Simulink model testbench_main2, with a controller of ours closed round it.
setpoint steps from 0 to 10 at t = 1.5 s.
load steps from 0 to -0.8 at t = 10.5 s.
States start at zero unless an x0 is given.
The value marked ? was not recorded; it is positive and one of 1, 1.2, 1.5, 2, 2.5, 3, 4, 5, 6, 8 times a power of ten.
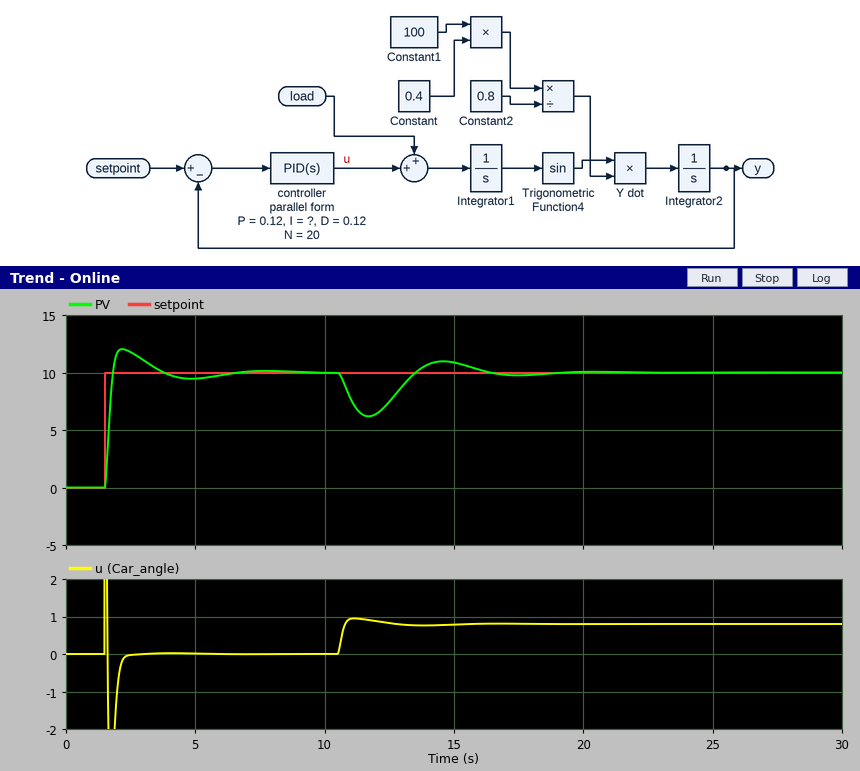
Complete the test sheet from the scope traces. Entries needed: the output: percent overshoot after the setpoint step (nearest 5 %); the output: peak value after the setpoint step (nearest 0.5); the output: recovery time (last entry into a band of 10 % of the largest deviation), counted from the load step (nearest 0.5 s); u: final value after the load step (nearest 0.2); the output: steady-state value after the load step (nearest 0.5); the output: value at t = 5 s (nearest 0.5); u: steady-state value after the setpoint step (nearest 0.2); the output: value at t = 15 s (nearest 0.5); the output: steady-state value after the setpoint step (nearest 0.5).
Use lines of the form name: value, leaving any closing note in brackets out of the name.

the output: percent overshoot after the setpoint step: 20 %
the output: peak value after the setpoint step: 12.0
the output: recovery time (last entry into a band of 10 % of the largest deviation), counted from the load step: 5.5 s
u: final value after the load step: 0.8
the output: steady-state value after the load step: 10.0
the output: value at t = 5 s: 9.5
u: steady-state value after the setpoint step: 0.0
the output: value at t = 15 s: 11.0
the output: steady-state value after the setpoint step: 10.0
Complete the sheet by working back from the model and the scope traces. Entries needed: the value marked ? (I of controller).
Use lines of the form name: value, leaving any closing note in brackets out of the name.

the value marked ?: 0.15
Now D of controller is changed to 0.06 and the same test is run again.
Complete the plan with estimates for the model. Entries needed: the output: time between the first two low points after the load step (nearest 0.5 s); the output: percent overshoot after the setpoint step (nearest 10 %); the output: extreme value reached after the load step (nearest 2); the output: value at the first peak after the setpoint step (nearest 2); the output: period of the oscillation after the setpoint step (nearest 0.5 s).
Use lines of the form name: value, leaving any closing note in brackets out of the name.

the output: time between the first two low points after the load step: 3.5 s
the output: percent overshoot after the setpoint step: 50 %
the output: extreme value reached after the load step: 4
the output: value at the first peak after the setpoint step: 14
the output: period of the oscillation after the setpoint step: 3.0 s
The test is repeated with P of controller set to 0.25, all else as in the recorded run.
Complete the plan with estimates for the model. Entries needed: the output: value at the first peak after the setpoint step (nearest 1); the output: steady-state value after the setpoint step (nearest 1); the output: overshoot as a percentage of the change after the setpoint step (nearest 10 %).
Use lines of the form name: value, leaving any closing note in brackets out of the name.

the output: value at the first peak after the setpoint step: 13
the output: steady-state value after the setpoint step: 10
the output: overshoot as a percentage of the change after the setpoint step: 30 %
